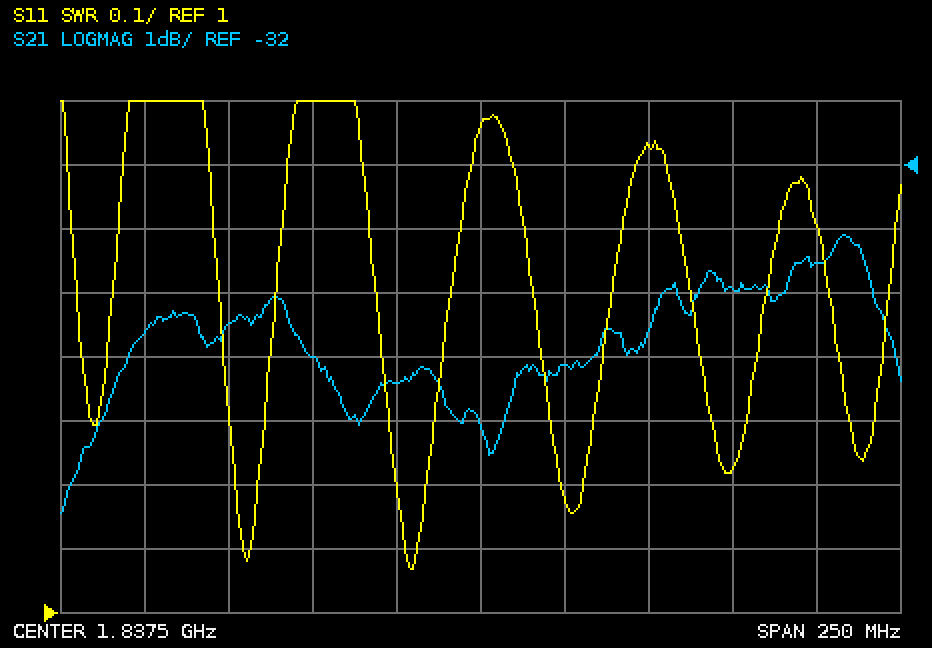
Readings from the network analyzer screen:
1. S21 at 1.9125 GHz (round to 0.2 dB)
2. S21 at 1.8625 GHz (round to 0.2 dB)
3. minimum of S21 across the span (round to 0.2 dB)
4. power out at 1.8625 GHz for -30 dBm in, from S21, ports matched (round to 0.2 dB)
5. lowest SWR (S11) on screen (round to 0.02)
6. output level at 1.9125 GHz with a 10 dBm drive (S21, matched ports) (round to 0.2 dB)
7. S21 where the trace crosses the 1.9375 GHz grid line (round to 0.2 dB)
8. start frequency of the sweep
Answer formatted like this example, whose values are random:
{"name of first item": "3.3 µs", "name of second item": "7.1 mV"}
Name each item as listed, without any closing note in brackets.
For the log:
{"S21 at 1.9125 GHz": "-34.0 dB", "S21 at 1.8625 GHz": "-35.2 dB", "minimum of S21 across the span": "-37.4 dB", "power out at 1.8625 GHz for -30 dBm in, from S21, ports matched": "-65.2 dBm", "lowest SWR (S11) on screen": "1.06", "output level at 1.9125 GHz with a 10 dBm drive (S21, matched ports)": "-24.0 dBm", "S21 where the trace crosses the 1.9375 GHz grid line": "-33.6 dB", "start frequency of the sweep": "1.7125 GHz"}
